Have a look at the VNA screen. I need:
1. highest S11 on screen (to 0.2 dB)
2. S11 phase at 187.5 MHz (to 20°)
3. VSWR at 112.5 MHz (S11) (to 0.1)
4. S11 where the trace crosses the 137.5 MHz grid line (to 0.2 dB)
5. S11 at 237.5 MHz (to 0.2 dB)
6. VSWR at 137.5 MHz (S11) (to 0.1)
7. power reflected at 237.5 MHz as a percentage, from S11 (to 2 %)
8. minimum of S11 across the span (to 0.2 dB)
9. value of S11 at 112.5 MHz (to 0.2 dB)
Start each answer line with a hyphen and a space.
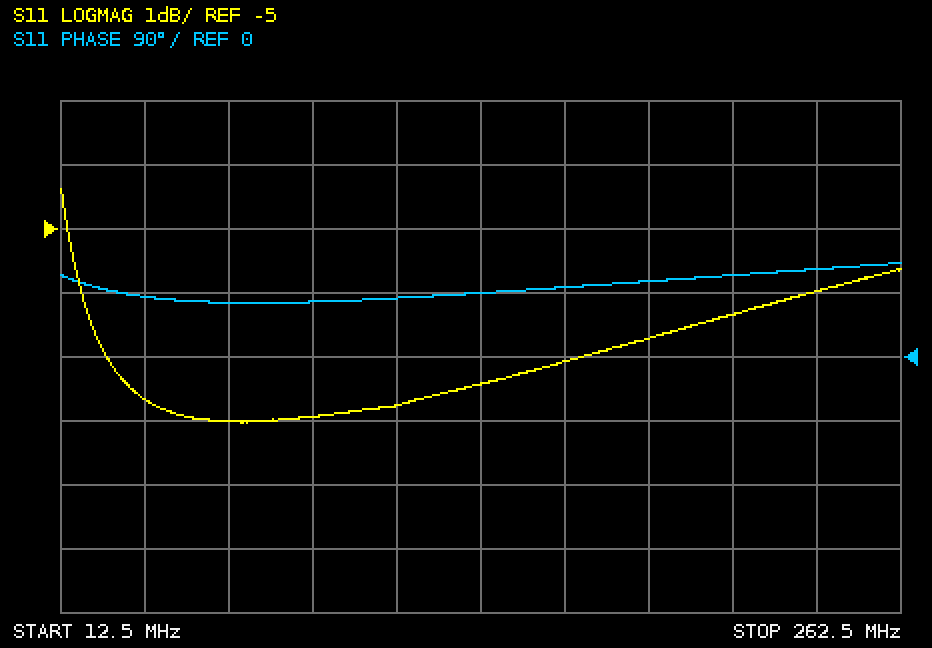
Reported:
- -4.4 dB
- 100°
- 2.4
- -7.4 dB
- -6.0 dB
- 2.5
- 26 %
- -8.0 dB
- -7.8 dB
